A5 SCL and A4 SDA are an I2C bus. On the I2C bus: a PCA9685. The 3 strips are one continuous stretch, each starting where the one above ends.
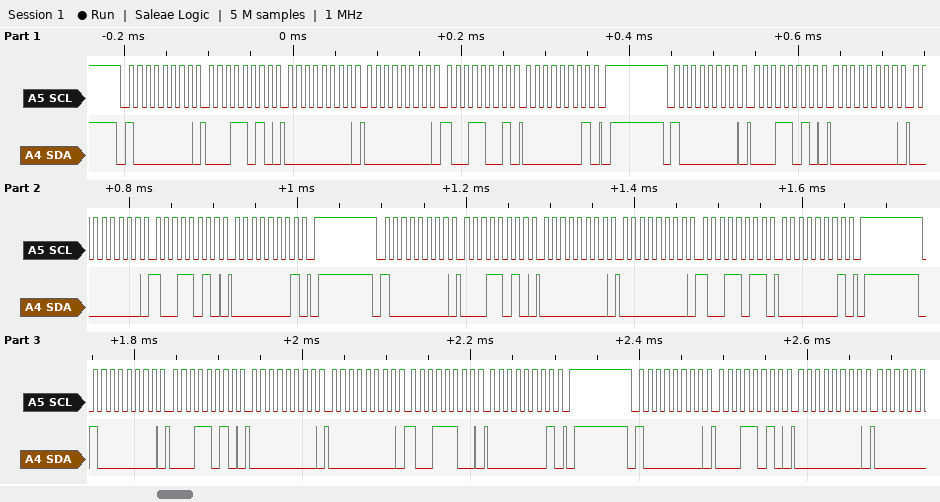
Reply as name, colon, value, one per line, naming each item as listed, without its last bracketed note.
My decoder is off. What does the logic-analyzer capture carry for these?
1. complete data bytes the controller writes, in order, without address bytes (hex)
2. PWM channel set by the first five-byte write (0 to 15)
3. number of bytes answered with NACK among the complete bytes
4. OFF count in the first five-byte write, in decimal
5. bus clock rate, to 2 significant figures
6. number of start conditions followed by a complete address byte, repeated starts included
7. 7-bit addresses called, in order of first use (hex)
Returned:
complete data bytes the controller writes, in order, without address bytes: 1A 00 00 99 01 1A 00 00 9A 01 1A 00 00 9B 01 1A 00 00 9C 01 1A 00
PWM channel set by the first five-byte write: 5
number of bytes answered with NACK among the complete bytes: 0
OFF count in the first five-byte write, in decimal: 409
bus clock rate, to 2 significant figures: 100 kHz
number of start conditions followed by a complete address byte, repeated starts included: 5
7-bit addresses called, in order of first use: 0x40
